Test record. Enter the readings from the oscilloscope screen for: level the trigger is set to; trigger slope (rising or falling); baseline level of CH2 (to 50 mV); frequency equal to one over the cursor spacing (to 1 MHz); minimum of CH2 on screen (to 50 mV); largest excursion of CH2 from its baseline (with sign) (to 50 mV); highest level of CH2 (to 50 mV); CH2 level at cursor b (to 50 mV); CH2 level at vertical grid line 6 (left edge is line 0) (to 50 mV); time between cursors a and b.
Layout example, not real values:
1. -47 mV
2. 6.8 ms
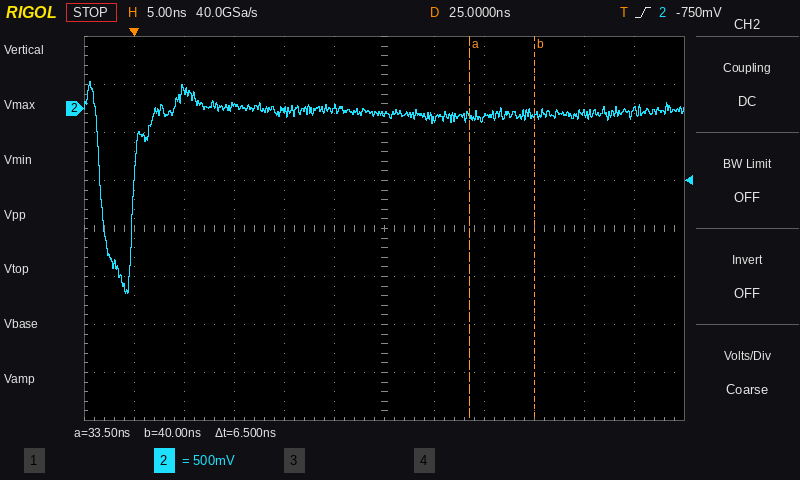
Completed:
1. -750 mV
2. rising
3. -50 mV
4. 154 MHz
5. -1.95 V
6. -1.90 V
7. 300 mV
8. -50 mV
9. -50 mV
10. 6.5 ns
